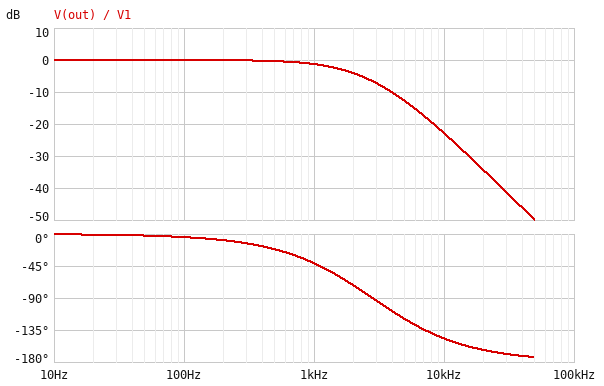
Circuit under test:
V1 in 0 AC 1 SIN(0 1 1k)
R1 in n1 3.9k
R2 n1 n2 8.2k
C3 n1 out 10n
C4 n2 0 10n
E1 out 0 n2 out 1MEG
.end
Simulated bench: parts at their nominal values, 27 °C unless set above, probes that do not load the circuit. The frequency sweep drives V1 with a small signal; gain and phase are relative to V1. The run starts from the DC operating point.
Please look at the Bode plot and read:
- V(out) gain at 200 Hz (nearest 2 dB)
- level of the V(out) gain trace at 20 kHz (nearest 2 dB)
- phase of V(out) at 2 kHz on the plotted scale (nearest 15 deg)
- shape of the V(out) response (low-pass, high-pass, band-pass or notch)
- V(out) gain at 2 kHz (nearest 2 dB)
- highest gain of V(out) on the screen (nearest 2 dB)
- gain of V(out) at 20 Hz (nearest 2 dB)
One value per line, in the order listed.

0 dB
-34 dB
-75 deg
low-pass
-4 dB
0 dB
0 dB
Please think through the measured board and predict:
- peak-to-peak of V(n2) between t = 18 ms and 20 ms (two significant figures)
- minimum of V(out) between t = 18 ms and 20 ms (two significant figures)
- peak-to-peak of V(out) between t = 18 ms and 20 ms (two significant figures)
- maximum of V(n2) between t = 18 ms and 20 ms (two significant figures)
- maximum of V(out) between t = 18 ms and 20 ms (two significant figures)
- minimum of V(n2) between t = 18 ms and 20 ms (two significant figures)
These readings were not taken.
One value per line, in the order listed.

1.7 V
-860 mV
1.7 V
860 mV
860 mV
-860 mV
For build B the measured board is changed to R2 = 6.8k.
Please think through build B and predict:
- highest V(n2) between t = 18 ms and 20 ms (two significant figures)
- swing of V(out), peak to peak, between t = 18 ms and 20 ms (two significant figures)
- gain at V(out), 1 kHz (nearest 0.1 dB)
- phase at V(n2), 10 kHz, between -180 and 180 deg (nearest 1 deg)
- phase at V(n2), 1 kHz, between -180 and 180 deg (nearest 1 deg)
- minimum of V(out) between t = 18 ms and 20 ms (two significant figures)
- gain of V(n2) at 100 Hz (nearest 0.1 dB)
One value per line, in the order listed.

890 mV
1.8 V
-1.0 dB
-145 deg
-37 deg
-890 mV
0 dB
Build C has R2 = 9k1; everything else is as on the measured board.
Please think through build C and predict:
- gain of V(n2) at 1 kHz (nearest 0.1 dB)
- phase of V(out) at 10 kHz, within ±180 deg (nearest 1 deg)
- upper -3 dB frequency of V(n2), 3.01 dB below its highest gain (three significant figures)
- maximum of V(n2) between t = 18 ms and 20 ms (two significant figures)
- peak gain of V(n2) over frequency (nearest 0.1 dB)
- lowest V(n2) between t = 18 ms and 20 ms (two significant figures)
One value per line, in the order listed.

-1.5 dB
-148 deg
1.52 kHz
840 mV
0 dB
-840 mV
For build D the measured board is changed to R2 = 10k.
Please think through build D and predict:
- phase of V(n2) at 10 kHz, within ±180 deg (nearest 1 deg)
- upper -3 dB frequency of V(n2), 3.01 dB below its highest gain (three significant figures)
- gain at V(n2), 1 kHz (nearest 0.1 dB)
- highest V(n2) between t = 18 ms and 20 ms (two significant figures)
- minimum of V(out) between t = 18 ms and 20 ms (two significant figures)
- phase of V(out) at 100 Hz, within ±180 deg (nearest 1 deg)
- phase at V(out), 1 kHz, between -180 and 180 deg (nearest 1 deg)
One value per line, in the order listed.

-149 deg
1.41 kHz
-1.7 dB
820 mV
-820 mV
-5 deg
-46 deg
